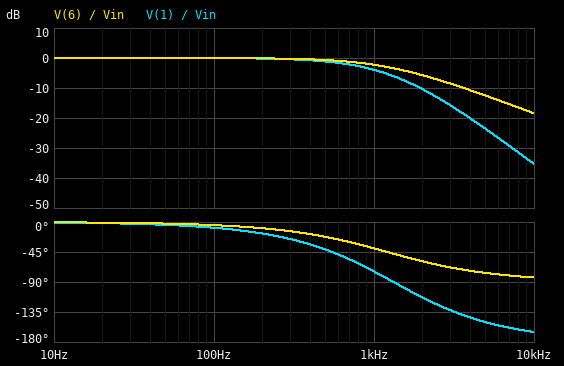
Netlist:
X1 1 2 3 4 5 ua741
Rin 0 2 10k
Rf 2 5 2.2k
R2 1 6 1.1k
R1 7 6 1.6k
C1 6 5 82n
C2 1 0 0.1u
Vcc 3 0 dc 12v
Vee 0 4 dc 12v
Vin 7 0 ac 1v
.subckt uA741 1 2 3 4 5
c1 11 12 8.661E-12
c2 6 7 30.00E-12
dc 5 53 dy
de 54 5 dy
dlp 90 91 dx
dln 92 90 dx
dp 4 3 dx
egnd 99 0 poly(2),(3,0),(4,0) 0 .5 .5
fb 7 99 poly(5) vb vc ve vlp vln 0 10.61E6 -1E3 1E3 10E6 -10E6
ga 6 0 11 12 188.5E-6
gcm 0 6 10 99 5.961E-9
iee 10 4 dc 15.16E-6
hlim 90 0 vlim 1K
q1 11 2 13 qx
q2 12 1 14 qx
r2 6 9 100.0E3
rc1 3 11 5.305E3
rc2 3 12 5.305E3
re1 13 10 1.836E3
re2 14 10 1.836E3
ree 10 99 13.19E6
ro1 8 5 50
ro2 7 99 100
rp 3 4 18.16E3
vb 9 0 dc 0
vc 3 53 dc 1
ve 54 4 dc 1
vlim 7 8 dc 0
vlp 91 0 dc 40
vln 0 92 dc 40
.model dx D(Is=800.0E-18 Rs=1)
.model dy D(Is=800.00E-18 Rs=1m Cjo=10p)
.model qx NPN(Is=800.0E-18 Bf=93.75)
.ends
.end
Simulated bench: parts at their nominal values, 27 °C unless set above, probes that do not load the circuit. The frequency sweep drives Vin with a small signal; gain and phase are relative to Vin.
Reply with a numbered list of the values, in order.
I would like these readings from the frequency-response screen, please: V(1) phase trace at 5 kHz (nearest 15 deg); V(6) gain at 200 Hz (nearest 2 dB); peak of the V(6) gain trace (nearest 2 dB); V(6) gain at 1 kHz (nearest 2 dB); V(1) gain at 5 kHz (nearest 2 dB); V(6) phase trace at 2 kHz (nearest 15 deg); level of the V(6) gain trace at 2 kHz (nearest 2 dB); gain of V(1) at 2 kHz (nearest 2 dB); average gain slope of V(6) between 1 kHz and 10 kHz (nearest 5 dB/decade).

1. -150 deg
2. 0 dB
3. 0 dB
4. -2 dB
5. -24 dB
6. -60 deg
7. -6 dB
8. -10 dB
9. -15 dB/decade
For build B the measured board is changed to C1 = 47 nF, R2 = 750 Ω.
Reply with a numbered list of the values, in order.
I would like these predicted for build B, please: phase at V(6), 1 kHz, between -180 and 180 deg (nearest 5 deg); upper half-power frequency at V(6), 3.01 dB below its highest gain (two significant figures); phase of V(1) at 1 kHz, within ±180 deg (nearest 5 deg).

1. -35 deg
2. 980 Hz
3. -60 deg
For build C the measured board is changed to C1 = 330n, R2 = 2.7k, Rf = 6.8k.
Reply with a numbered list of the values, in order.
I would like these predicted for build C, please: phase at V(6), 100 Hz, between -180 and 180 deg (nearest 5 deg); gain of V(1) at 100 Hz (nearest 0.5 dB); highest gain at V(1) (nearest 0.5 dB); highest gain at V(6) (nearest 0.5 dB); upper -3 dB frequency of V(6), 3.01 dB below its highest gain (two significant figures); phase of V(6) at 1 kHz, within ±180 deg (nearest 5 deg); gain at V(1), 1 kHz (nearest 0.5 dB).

1. 5 deg
2. 0.5 dB
3. 14.5 dB
4. 16.5 dB
5. 460 Hz
6. -115 deg
7. -13.5 dB
